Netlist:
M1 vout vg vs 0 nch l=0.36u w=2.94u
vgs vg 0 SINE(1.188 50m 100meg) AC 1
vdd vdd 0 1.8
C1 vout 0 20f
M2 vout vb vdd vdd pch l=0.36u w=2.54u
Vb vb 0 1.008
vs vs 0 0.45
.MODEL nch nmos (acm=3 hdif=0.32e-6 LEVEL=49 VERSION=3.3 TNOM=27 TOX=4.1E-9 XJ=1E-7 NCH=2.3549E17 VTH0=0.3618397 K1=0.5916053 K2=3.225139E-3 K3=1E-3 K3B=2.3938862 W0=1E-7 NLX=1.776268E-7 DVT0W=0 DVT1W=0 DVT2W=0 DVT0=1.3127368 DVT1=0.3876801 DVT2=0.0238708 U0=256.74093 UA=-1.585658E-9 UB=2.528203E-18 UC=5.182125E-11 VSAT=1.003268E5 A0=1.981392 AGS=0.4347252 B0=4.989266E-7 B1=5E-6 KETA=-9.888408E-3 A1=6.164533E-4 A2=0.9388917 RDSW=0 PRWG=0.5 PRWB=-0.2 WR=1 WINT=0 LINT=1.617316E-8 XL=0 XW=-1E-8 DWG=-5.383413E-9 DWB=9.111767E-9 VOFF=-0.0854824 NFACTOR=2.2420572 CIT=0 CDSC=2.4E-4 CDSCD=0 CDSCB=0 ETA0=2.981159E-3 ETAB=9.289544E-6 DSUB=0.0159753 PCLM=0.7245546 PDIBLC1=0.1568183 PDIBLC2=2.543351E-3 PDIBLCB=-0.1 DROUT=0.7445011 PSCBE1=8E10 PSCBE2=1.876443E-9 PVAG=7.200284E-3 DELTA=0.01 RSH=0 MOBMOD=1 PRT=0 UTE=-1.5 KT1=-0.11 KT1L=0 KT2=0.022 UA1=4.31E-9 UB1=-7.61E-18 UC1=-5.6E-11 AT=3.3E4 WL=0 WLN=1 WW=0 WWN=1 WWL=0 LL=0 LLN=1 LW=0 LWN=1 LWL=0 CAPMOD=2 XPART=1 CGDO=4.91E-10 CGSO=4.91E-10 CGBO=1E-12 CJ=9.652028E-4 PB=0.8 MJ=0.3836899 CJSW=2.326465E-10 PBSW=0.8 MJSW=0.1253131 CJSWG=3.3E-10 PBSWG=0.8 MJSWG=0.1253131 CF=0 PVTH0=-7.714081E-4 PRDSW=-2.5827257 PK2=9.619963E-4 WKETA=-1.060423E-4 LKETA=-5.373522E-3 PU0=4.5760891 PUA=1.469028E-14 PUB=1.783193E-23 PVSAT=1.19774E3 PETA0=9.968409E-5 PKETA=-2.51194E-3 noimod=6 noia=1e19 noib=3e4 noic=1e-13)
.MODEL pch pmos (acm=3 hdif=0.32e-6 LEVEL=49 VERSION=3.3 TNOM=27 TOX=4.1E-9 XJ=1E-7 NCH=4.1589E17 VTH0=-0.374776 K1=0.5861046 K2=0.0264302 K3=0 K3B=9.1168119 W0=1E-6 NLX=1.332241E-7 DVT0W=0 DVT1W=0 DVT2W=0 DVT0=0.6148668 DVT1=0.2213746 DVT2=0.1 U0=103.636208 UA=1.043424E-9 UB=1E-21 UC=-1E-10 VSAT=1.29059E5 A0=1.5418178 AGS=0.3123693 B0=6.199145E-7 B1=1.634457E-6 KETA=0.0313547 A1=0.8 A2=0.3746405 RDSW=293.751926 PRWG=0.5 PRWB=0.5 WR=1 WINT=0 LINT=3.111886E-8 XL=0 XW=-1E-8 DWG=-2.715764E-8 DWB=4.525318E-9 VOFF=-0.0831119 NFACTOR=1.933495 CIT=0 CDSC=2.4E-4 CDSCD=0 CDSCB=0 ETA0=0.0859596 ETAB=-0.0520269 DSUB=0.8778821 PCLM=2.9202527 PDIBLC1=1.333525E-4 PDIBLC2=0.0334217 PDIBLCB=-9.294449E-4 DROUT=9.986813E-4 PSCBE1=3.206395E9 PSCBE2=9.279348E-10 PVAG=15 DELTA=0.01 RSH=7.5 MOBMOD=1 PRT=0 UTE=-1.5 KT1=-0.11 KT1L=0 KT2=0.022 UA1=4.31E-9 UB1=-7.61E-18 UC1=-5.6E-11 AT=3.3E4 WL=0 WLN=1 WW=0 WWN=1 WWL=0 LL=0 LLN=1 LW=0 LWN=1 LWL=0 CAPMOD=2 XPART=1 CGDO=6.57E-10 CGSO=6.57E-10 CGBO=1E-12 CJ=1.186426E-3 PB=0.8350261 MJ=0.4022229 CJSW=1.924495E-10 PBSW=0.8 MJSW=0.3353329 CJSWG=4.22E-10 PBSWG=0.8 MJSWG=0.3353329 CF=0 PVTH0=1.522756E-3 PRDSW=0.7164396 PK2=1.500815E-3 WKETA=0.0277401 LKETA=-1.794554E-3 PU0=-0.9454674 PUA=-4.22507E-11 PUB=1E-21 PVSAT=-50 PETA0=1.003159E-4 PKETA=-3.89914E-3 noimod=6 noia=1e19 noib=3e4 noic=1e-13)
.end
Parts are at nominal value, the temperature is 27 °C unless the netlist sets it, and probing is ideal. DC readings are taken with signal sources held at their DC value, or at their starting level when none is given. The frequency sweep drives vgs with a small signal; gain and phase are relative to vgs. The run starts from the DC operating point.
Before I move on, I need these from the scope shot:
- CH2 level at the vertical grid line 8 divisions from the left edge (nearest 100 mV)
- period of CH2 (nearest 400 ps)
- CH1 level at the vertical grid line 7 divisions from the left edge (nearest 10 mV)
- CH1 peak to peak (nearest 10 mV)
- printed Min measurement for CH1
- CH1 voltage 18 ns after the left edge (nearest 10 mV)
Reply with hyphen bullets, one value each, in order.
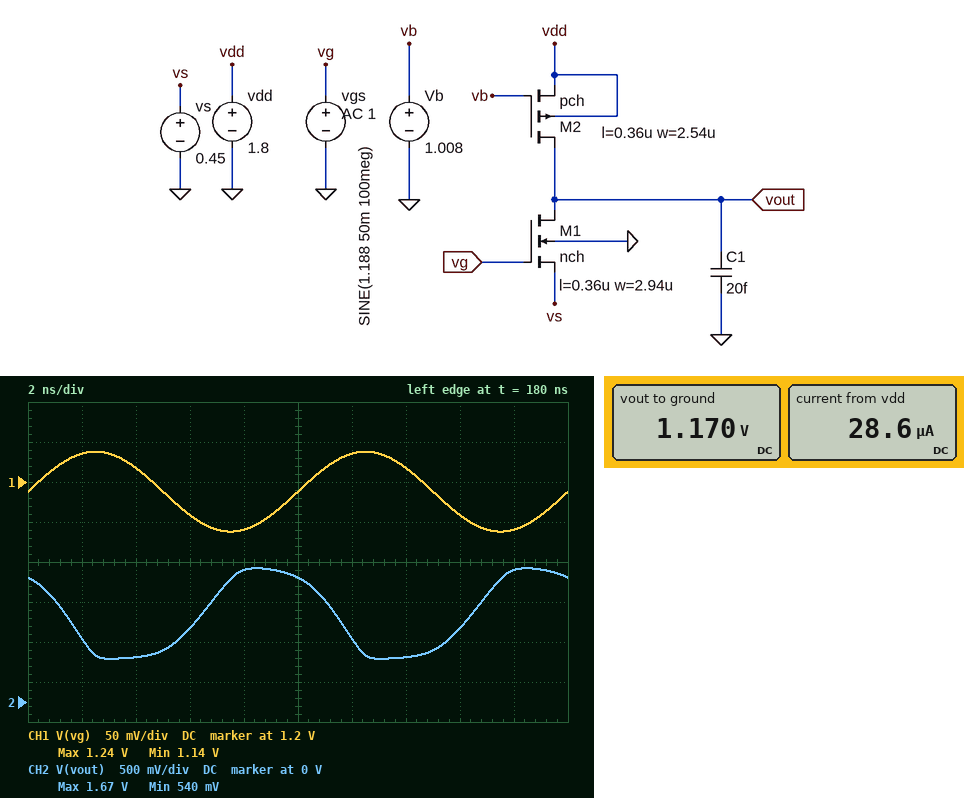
- 900 mV
- 10.0 ns
- 1.22 V
- 100 mV
- 1.14 V
- 1.14 V
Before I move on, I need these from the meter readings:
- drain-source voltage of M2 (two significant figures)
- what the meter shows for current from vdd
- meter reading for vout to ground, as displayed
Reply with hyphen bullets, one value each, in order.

- -630 mV
- 28.6 µA
- 1.170 V
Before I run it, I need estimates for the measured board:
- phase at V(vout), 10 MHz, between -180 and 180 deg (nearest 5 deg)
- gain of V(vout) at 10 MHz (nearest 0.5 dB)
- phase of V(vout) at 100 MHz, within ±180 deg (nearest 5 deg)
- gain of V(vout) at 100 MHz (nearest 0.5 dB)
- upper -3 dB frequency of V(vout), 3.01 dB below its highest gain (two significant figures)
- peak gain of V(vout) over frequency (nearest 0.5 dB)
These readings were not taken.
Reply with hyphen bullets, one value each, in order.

- 170 deg
- 32.0 dB
- 115 deg
- 24.5 dB
- 47 MHz
- 32.0 dB
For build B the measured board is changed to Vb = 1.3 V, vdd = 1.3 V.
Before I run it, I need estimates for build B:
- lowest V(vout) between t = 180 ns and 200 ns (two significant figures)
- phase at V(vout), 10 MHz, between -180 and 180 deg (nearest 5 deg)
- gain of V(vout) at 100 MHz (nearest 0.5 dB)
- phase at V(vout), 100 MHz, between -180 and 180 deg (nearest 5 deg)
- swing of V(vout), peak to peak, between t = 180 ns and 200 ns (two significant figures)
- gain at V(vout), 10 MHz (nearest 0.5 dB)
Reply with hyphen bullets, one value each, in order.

- 450 mV
- 90 deg
- -40.0 dB
- 85 deg
- 1.1 mV
- -60.0 dB
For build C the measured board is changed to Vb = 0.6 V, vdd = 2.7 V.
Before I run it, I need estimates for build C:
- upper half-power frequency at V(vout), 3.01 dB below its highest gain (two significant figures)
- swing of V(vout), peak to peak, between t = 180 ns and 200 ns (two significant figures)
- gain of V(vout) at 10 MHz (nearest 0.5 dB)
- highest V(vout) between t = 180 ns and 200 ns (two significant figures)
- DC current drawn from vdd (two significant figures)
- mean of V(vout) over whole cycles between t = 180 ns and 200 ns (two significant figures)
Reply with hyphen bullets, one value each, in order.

- 2.6 GHz
- 60 mV
- -4.5 dB
- 2.7 V
- 35 µA
- 2.6 V
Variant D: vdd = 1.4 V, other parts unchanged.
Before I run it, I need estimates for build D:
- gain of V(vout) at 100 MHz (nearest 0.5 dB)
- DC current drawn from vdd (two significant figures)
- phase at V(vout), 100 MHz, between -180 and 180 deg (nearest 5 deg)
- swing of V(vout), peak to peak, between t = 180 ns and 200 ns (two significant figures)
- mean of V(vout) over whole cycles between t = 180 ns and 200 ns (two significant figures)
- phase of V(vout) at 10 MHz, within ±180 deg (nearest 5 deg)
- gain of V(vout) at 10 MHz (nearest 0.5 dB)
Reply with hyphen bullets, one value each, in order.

- -39.5 dB
- 130 nA
- 105 deg
- 1.1 mV
- 450 mV
- 160 deg
- -50.0 dB
